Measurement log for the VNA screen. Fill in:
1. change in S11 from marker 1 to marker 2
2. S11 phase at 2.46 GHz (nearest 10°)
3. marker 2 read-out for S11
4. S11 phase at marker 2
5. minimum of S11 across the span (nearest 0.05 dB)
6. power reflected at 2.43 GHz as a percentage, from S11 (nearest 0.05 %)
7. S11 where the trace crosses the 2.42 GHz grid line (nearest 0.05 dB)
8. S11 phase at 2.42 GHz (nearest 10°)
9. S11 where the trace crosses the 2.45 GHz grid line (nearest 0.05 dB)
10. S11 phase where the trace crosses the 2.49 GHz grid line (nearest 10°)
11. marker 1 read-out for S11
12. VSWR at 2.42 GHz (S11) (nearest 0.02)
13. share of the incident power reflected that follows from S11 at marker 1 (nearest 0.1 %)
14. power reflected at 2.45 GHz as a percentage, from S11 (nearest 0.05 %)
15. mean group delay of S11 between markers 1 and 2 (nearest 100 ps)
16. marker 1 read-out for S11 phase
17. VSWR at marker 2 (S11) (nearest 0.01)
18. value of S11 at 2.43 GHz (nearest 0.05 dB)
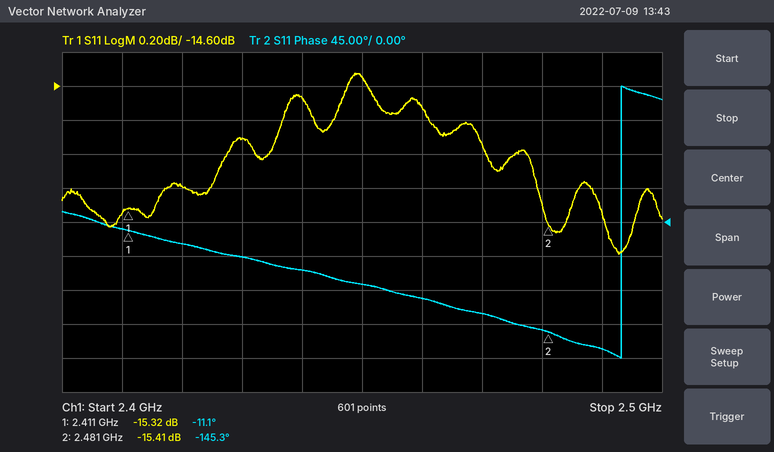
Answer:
-0.09 dB
-100°
-15.41 dB
-145.3°
-15.60 dB
3.25 %
-15.20 dB
-30°
-14.55 dB
-170°
-15.32 dB
1.42
2.9 %
3.50 %
5.3 ns
-11.1°
1.41
-14.90 dB
